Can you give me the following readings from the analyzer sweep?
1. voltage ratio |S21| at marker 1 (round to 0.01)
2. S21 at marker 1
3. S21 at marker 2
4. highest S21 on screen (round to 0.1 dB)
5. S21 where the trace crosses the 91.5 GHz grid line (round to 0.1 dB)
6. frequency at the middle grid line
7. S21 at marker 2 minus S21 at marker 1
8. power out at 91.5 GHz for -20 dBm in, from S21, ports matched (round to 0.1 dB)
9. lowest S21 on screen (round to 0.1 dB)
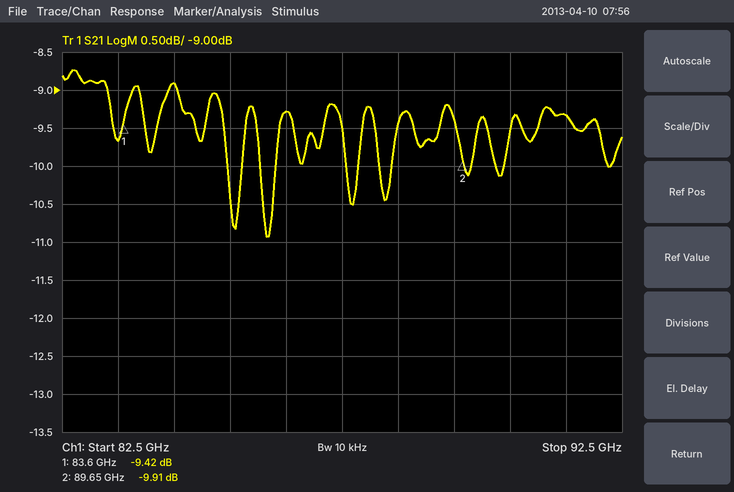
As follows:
0.34
-9.42 dB
-9.91 dB
-8.7 dB
-9.3 dB
87.5 GHz
-0.49 dB
-29.3 dBm
-10.9 dB
